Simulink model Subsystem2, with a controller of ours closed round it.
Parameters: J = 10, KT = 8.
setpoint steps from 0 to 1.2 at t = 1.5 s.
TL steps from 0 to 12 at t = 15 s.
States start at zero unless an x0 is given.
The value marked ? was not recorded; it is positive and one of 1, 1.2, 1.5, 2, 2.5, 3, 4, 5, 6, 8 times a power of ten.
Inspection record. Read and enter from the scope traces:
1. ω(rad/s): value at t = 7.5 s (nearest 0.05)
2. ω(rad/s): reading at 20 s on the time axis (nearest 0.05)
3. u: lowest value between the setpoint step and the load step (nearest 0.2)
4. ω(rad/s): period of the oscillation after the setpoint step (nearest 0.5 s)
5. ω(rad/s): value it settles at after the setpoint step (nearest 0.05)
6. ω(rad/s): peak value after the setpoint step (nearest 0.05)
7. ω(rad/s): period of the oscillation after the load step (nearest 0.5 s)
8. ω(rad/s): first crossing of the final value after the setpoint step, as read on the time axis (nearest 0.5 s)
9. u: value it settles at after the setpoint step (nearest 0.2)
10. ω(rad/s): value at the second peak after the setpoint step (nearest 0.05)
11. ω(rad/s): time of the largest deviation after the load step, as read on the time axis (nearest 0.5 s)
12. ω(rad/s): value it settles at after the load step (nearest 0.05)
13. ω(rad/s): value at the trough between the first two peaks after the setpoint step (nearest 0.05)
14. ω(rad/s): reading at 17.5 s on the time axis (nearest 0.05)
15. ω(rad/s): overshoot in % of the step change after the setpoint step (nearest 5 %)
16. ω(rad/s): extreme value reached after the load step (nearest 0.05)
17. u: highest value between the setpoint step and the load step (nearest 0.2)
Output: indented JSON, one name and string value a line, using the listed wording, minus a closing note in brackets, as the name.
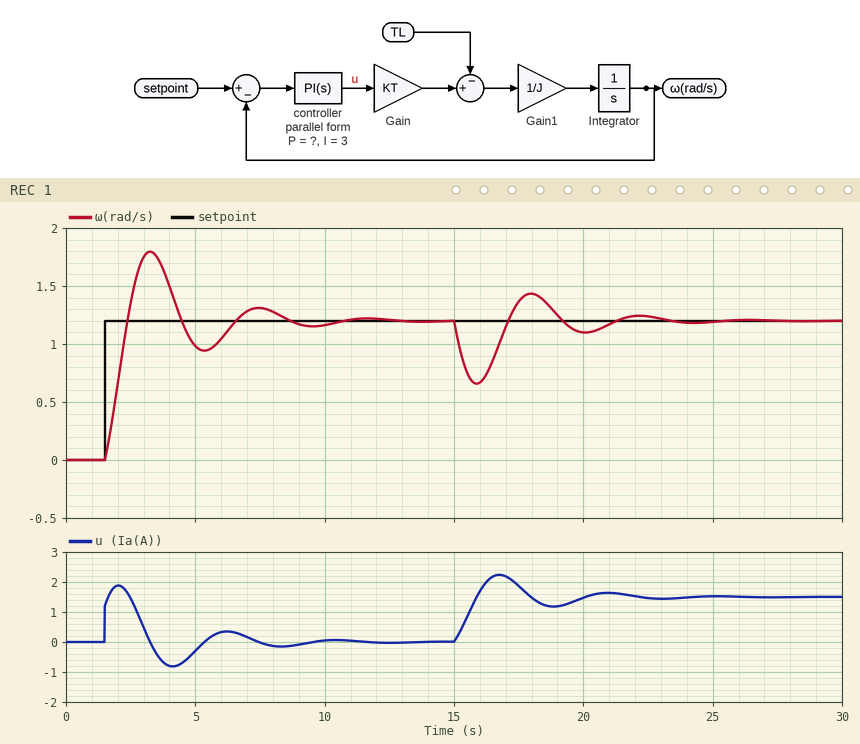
{
  "ω(rad/s): value at t = 7.5 s": "1.30",
  "ω(rad/s): reading at 20 s on the time axis": "1.10",
  "u: lowest value between the setpoint step and the load step": "-0.8",
  "ω(rad/s): period of the oscillation after the setpoint step": "4.0 s",
  "ω(rad/s): value it settles at after the setpoint step": "1.20",
  "ω(rad/s): peak value after the setpoint step": "1.80",
  "ω(rad/s): period of the oscillation after the load step": "4.0 s",
  "ω(rad/s): first crossing of the final value after the setpoint step, as read on the time axis": "2.5 s",
  "u: value it settles at after the setpoint step": "0.0",
  "ω(rad/s): value at the second peak after the setpoint step": "1.30",
  "ω(rad/s): time of the largest deviation after the load step, as read on the time axis": "16.0 s",
  "ω(rad/s): value it settles at after the load step": "1.20",
  "ω(rad/s): value at the trough between the first two peaks after the setpoint step": "0.95",
  "ω(rad/s): reading at 17.5 s on the time axis": "1.35",
  "ω(rad/s): overshoot in % of the step change after the setpoint step": "50 %",
  "ω(rad/s): extreme value reached after the load step": "0.65",
  "u: highest value between the setpoint step and the load step": "1.8"
}
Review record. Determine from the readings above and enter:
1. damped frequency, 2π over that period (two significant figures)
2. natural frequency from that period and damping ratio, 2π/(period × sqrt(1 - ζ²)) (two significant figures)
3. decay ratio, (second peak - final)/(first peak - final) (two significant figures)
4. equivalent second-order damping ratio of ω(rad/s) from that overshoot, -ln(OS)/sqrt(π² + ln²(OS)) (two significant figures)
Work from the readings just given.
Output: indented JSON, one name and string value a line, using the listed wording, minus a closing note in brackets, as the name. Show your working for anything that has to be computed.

{
  "damped frequency, 2π over that period": "2π / 4 = 1.6 rad/s",
  "natural frequency from that period and damping ratio, 2π/(period × sqrt(1 - ζ²))": "2π / (4 × sqrt(1 - 0.22²)) = 1.6 rad/s",
  "decay ratio, (second peak - final)/(first peak - final)": "(1.3 - 1.2) / (1.8 - 1.2) = 0.17",
  "equivalent second-order damping ratio of ω(rad/s) from that overshoot, -ln(OS)/sqrt(π² + ln²(OS))": "ln(0.5) = -0.693; 0.693 / sqrt(9.870 + 0.480) = 0.22"
}
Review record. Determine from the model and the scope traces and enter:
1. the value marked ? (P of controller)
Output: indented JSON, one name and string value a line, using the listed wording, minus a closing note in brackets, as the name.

{
  "the value marked ?": "1"
}
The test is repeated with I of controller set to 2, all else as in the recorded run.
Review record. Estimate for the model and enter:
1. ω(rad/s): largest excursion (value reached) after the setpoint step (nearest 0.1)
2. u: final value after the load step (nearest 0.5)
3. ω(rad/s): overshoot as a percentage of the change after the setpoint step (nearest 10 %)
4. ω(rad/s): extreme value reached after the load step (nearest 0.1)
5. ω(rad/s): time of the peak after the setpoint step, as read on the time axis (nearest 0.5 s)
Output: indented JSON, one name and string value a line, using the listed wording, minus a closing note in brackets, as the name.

{
  "ω(rad/s): largest excursion (value reached) after the setpoint step": "1.7",
  "u: final value after the load step": "1.5",
  "ω(rad/s): overshoot as a percentage of the change after the setpoint step": "40 %",
  "ω(rad/s): extreme value reached after the load step": "0.6",
  "ω(rad/s): time of the peak after the setpoint step, as read on the time axis": "3.5 s"
}
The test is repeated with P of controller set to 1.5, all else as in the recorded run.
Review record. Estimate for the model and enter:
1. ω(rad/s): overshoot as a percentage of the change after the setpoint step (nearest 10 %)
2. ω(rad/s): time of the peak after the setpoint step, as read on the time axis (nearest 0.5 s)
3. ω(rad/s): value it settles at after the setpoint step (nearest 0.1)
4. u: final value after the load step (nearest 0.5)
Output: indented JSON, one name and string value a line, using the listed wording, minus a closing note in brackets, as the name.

{
  "ω(rad/s): overshoot as a percentage of the change after the setpoint step": "40 %",
  "ω(rad/s): time of the peak after the setpoint step, as read on the time axis": "3.0 s",
  "ω(rad/s): value it settles at after the setpoint step": "1.2",
  "u: final value after the load step": "1.5"
}
